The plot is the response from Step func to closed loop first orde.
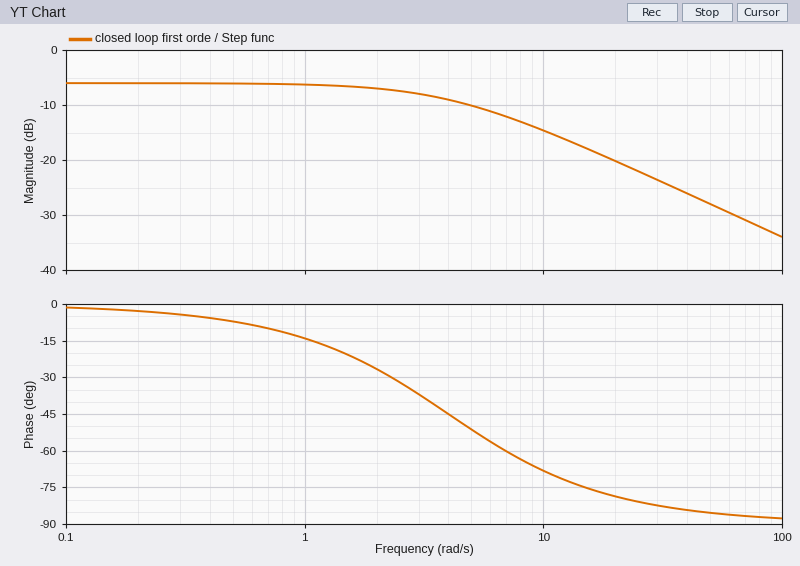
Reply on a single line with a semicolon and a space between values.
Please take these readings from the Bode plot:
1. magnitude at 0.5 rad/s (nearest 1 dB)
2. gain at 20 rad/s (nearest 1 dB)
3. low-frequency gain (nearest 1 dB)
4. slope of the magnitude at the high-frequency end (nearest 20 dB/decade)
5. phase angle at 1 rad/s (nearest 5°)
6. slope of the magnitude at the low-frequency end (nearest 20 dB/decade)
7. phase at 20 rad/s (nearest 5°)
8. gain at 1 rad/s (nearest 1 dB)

-6 dB; -20 dB; -6 dB; -20 dB/decade; -15°; 0 dB/decade; -80°; -6 dB
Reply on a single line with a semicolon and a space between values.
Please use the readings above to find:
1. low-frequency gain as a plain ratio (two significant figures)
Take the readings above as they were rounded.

0.50
